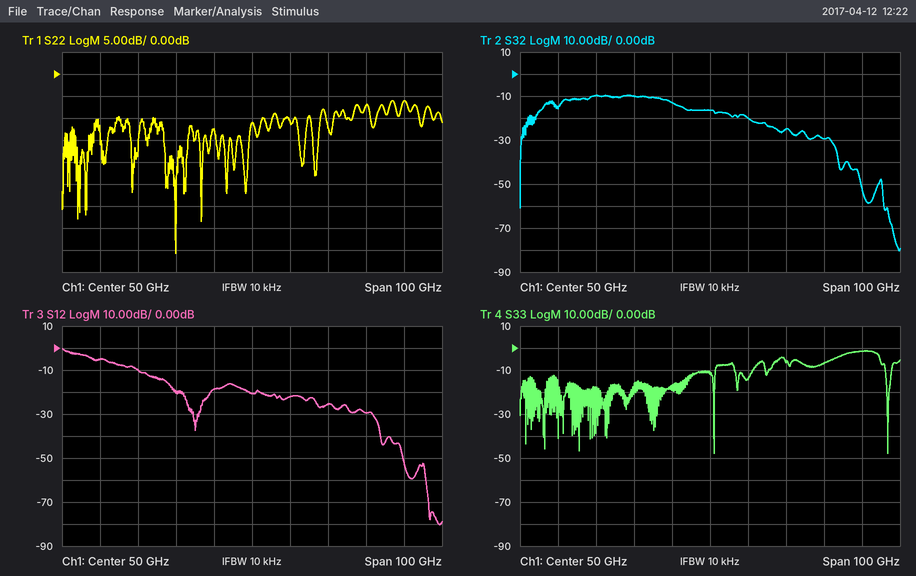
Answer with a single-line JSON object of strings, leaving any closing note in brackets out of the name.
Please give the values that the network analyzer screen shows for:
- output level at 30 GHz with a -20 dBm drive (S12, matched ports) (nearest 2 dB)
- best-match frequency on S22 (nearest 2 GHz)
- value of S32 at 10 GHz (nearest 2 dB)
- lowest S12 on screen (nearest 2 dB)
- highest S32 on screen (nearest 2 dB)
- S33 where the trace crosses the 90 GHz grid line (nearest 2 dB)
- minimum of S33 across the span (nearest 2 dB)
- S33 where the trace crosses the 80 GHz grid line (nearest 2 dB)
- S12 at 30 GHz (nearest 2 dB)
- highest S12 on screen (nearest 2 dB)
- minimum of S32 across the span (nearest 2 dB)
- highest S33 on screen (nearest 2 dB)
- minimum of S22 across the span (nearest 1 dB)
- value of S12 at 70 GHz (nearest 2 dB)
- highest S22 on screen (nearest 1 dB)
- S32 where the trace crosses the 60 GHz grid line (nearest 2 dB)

{"output level at 30 GHz with a -20 dBm drive (S12, matched ports)": "-40 dBm", "best-match frequency on S22": "30 GHz", "value of S32 at 10 GHz": "-16 dB", "lowest S12 on screen": "-80 dB", "highest S32 on screen": "-10 dB", "S33 where the trace crosses the 90 GHz grid line": "-2 dB", "minimum of S33 across the span": "-48 dB", "S33 where the trace crosses the 80 GHz grid line": "-6 dB", "S12 at 30 GHz": "-20 dB", "highest S12 on screen": "0 dB", "minimum of S32 across the span": "-80 dB", "highest S33 on screen": "-2 dB", "minimum of S22 across the span": "-41 dB", "value of S12 at 70 GHz": "-26 dB", "highest S22 on screen": "-6 dB", "S32 where the trace crosses the 60 GHz grid line": "-20 dB"}
